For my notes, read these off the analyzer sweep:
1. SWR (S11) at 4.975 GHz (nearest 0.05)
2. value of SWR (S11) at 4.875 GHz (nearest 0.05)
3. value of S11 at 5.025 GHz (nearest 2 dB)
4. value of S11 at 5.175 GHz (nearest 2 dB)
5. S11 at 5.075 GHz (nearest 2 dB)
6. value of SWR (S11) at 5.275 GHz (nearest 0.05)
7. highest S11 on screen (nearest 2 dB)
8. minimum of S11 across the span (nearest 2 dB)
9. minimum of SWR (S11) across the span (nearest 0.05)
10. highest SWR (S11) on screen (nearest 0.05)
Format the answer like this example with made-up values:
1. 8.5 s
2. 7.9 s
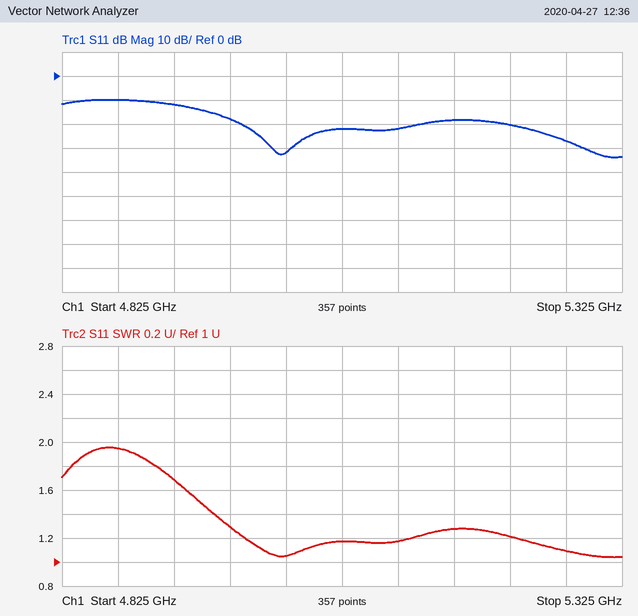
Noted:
1. 1.30
2. 1.95
3. -32 dB
4. -18 dB
5. -22 dB
6. 1.10
7. -10 dB
8. -34 dB
9. 1.05
10. 1.95
